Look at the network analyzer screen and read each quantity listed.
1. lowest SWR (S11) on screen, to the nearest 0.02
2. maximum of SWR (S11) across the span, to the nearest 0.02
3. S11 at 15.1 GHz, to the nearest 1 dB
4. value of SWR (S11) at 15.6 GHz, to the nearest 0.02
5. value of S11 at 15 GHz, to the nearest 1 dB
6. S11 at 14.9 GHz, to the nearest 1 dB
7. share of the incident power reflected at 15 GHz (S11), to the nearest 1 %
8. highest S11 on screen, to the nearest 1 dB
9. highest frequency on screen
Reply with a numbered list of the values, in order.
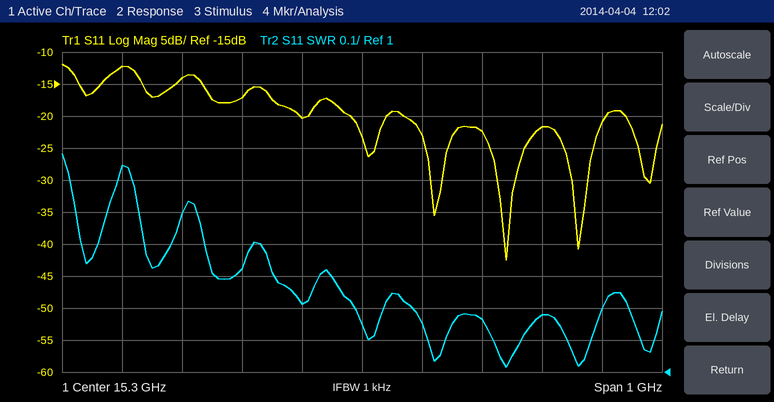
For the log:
1. 1.02
2. 1.68
3. -17 dB
4. 1.18
5. -14 dB
6. -12 dB
7. 4 %
8. -12 dB
9. 15.8 GHz
